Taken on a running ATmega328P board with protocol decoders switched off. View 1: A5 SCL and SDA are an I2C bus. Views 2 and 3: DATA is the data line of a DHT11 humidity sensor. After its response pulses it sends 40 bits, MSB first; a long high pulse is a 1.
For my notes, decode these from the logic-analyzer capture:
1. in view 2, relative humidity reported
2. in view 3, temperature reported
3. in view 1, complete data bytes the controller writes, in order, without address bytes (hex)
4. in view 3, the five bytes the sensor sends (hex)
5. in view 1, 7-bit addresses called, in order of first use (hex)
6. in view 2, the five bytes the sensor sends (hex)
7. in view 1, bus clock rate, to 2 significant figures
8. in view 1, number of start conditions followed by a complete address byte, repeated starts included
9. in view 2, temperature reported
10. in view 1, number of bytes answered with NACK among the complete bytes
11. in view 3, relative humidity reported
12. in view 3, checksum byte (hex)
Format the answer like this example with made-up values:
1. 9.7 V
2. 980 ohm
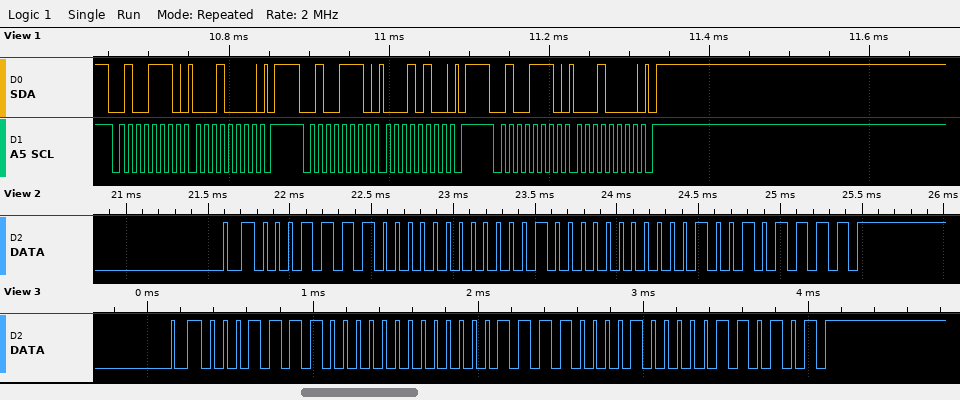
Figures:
1. 30 %
2. 15.8 °C
3. 10 14 10
4. 1E 00 0F 08 35
5. 0x27
6. 1E 00 10 01 2F
7. 100 kHz
8. 3
9. 16.1 °C
10. 0
11. 30 %
12. 0x35
